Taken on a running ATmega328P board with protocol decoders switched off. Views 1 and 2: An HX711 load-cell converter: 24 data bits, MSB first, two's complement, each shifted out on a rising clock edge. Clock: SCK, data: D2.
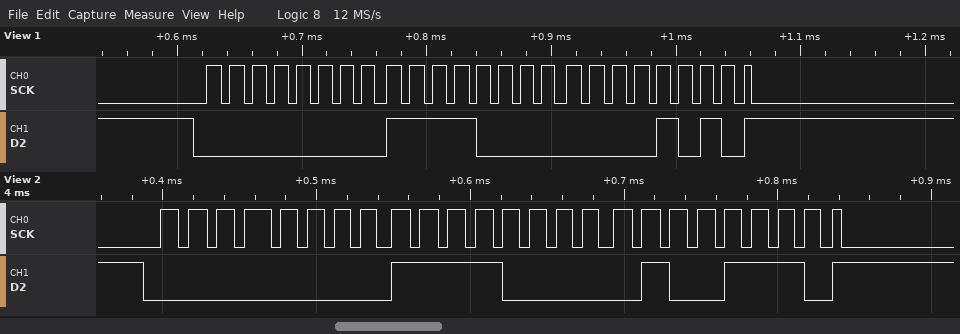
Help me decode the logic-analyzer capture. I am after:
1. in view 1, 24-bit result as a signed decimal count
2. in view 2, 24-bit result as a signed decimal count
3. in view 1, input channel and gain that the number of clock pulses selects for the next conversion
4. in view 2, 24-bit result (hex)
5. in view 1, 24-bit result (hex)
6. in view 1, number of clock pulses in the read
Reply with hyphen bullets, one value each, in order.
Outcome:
- 61450
- 61518
- channel A, gain 128
- 0x00F04E
- 0x00F00A
- 25
